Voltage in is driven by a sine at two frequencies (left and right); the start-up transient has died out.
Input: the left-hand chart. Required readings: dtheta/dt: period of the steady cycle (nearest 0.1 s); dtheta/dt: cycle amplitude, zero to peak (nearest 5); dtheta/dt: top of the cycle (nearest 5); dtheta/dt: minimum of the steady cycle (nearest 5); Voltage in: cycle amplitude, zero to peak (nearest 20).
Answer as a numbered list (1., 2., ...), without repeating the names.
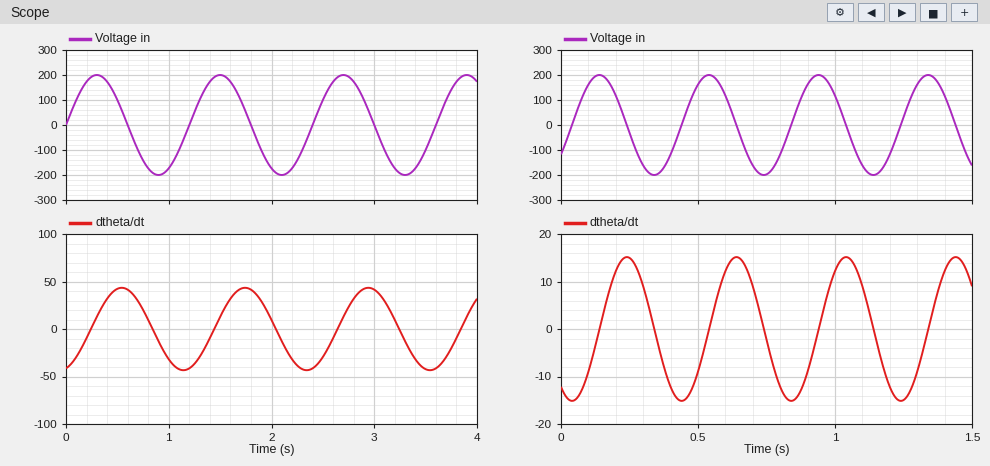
1. 1.2 s
2. 45
3. 45
4. -45
5. 200
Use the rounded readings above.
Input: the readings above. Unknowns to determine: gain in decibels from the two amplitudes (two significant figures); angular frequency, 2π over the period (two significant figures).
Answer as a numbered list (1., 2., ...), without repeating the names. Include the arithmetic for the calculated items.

1. 20 log10(45 / 200) = -13 dB
2. 2π / 1.2 = 5.2 rad/s
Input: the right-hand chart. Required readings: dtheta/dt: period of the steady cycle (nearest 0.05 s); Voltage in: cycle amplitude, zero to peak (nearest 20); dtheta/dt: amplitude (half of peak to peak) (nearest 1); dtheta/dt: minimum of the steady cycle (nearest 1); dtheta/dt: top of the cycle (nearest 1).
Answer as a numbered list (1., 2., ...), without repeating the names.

1. 0.40 s
2. 200
3. 15
4. -15
5. 15
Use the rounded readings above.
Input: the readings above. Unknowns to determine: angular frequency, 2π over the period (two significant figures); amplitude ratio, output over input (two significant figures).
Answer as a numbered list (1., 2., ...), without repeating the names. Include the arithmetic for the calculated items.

1. 2π / 0.4 = 16 rad/s
2. 15 / 200 = 0.075
